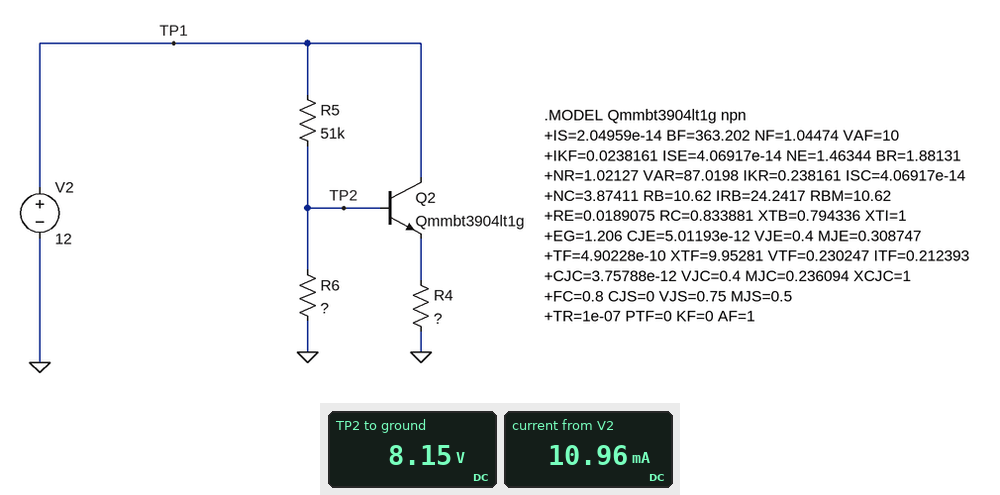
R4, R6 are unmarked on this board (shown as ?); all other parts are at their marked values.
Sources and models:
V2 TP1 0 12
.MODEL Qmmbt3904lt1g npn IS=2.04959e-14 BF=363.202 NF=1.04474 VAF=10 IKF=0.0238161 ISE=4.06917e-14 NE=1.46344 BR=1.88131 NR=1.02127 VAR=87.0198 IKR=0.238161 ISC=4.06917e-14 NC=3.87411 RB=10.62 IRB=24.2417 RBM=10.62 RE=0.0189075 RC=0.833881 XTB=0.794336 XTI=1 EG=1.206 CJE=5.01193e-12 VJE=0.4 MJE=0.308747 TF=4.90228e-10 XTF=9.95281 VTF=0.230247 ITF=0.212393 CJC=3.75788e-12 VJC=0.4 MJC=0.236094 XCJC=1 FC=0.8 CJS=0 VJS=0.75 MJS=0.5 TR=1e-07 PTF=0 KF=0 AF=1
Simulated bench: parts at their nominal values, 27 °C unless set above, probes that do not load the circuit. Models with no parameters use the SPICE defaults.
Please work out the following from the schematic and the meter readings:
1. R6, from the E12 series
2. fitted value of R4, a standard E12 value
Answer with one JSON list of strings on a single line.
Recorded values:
["220 kΩ", "680 Ω"]
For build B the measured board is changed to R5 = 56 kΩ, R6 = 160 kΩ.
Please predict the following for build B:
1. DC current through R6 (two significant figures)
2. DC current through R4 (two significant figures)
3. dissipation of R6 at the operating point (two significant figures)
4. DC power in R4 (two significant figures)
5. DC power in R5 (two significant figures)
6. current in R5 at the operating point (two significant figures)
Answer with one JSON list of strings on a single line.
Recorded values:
["47 µA", "10 mA", "350 µW", "68 mW", "360 µW", "80 µA"]
